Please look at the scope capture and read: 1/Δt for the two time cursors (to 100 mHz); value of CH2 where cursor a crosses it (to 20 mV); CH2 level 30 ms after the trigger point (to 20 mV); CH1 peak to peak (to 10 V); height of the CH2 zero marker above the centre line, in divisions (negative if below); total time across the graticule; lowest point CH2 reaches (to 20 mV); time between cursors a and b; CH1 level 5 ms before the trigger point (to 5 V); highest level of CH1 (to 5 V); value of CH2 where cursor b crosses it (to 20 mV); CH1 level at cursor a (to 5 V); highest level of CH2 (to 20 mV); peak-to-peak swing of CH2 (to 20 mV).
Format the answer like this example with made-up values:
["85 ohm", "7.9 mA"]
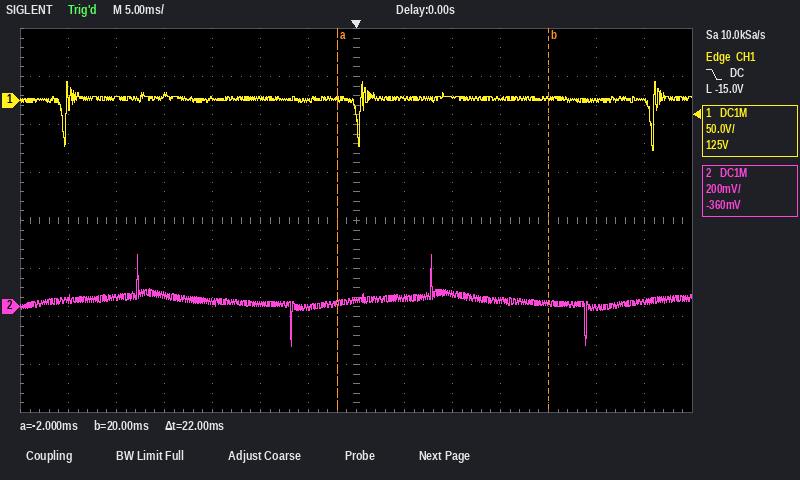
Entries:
["45.5 Hz", "20 mV", "20 mV", "70 V", "-1.8 div", "70 ms", "-160 mV", "22 ms", "0 V", "20 V", "20 mV", "0 V", "220 mV", "380 mV"]
